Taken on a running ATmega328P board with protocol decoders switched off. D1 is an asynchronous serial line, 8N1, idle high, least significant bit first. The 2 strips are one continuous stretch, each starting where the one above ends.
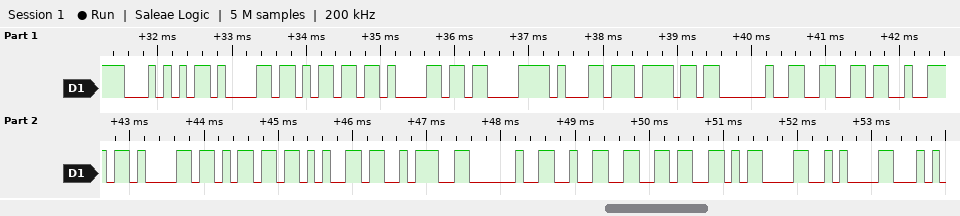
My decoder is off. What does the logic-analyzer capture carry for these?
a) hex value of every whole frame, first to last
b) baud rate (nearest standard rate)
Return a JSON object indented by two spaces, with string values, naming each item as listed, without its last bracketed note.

{
  "hex value of every whole frame, first to last": "0x54 0x61 0x6D 0x61 0xC3 0xB1 0x6F 0x20 0x66 0x72 0x61 0x6D 0x65 0x3A 0x20 0x32 0x36 0x0D 0x0A",
  "baud rate": "9600 baud"
}
